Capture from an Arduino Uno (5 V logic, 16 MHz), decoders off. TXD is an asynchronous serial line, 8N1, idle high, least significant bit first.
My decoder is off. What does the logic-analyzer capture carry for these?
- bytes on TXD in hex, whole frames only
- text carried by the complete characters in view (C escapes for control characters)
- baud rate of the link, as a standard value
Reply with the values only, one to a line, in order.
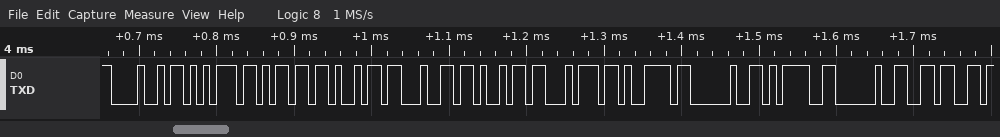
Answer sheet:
0x48 0x75 0x6D 0x69 0x64 0x69 0x74 0x79 0x20 0x3D 0x20 0x36
"Humidity = 6"
115200 baud
